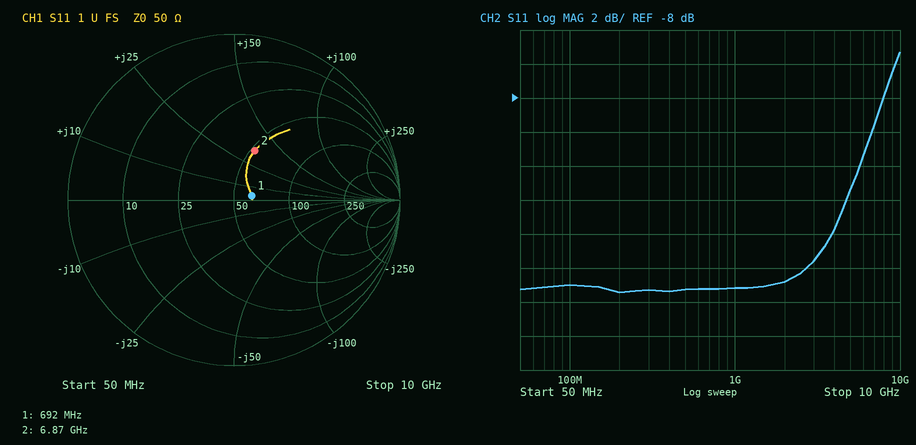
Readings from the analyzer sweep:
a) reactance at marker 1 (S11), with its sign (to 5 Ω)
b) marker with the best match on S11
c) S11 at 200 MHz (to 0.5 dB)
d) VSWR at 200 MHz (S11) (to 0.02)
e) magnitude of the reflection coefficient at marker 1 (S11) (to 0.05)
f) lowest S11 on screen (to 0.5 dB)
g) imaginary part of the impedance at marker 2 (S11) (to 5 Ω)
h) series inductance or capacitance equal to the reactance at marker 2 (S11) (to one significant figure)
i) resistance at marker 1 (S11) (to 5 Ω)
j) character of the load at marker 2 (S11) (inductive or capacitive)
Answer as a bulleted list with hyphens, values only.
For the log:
- +5 Ω
- marker 1
- -19.5 dB
- 1.24
- 0.10
- -19.5 dB
- +35 Ω
- 800 pH
- 60 Ω
- inductive
